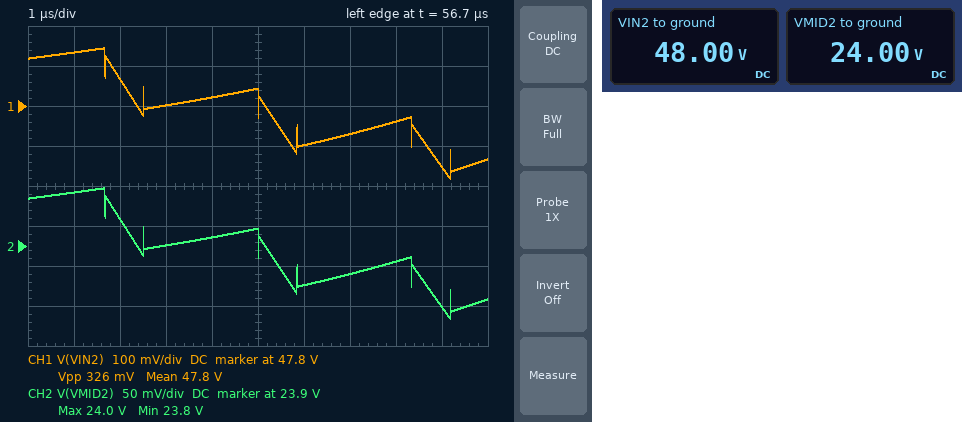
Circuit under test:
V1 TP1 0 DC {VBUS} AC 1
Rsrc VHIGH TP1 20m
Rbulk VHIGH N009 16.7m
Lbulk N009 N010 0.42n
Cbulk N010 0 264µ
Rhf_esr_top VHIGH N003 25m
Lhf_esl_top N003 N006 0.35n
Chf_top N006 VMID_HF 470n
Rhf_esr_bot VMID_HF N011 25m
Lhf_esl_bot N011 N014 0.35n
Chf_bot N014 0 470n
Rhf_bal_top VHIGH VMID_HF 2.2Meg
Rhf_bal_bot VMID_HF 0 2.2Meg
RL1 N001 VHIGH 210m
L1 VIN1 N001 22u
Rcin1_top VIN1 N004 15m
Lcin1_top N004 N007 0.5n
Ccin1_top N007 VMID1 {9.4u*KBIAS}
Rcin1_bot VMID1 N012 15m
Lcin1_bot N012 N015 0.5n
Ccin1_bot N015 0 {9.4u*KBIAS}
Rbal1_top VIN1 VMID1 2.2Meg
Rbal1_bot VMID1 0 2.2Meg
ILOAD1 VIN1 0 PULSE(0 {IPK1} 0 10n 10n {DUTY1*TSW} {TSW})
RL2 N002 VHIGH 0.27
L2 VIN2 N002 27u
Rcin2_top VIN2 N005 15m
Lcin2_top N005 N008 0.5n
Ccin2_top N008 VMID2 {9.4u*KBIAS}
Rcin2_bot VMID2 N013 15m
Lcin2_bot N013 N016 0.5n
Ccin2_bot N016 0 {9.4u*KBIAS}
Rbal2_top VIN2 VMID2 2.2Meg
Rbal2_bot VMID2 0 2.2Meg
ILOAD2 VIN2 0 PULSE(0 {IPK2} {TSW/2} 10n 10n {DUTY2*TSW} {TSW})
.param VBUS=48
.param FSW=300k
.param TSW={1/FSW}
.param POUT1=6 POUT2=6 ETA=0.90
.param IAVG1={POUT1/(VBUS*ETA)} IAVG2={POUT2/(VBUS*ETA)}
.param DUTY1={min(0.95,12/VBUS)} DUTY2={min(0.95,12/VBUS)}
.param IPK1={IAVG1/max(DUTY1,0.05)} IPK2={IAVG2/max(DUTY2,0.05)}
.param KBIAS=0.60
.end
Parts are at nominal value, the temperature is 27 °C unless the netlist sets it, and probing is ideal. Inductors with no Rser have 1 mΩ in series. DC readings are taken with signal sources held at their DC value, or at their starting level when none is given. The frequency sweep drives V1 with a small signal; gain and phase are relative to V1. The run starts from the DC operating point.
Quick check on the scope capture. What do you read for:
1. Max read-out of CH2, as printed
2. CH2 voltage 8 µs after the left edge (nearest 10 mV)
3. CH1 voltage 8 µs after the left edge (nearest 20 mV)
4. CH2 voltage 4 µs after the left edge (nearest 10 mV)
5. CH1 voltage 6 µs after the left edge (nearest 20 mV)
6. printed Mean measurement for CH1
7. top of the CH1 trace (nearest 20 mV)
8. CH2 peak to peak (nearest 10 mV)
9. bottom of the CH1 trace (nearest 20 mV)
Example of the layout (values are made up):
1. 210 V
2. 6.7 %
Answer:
1. 24.0 V
2. 23.88 V
3. 47.76 V
4. 23.91 V
5. 47.70 V
6. 47.8 V
7. 47.94 V
8. 160 mV
9. 47.62 V
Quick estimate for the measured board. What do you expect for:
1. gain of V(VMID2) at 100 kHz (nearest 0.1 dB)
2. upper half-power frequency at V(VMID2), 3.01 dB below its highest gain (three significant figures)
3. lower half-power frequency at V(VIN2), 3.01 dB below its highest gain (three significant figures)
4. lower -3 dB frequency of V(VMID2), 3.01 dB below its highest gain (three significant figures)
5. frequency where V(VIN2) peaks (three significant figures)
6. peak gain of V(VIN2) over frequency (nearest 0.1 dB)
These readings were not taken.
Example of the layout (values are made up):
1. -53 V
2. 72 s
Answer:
1. -41.5 dB
2. 19.1 kHz
3. 17.2 kHz
4. 17.2 kHz
5. 18.2 kHz
6. 17.1 dB
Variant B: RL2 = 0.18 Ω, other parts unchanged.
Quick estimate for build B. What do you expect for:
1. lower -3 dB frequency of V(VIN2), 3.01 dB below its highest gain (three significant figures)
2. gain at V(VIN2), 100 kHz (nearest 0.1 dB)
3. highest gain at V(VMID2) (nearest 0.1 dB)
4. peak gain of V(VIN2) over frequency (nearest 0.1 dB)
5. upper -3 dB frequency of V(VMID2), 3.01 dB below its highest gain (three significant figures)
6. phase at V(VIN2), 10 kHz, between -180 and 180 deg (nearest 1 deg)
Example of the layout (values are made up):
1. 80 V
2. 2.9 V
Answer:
1. 17.5 kHz
2. -35.5 dB
3. 14.0 dB
4. 20.0 dB
5. 18.9 kHz
6. -19 deg
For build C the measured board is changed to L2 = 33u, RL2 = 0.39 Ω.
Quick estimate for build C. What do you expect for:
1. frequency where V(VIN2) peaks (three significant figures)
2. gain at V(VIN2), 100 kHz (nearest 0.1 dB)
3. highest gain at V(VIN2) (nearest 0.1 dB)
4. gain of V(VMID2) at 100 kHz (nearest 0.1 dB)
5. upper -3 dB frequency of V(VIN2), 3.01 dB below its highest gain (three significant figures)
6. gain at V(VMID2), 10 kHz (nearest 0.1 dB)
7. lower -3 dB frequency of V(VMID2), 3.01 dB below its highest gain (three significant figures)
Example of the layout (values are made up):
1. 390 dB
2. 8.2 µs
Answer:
1. 16.4 kHz
2. -37.3 dB
3. 15.6 dB
4. -43.3 dB
5. 17.4 kHz
6. -3.2 dB
7. 15.3 kHz
